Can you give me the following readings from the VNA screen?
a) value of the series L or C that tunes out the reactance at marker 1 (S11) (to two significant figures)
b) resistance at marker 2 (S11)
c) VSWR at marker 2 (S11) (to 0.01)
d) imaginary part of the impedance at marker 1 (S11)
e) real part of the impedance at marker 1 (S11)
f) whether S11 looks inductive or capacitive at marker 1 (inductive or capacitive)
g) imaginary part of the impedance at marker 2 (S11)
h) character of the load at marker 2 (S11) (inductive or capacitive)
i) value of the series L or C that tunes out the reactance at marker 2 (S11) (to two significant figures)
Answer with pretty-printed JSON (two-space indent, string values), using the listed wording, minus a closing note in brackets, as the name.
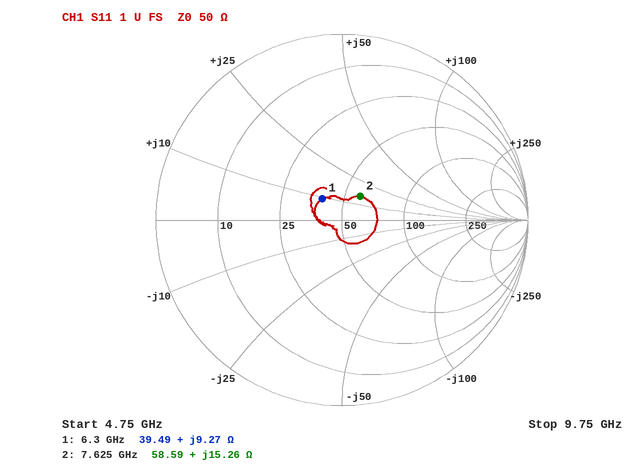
{
  "value of the series L or C that tunes out the reactance at marker 1 (S11)": "2.7 pF",
  "resistance at marker 2": "58.59 Ω",
  "VSWR at marker 2 (S11)": "1.38",
  "imaginary part of the impedance at marker 1": "+9.27 Ω",
  "real part of the impedance at marker 1": "39.49 Ω",
  "whether S11 looks inductive or capacitive at marker 1": "inductive",
  "imaginary part of the impedance at marker 2": "+15.26 Ω",
  "character of the load at marker 2 (S11)": "inductive",
  "value of the series L or C that tunes out the reactance at marker 2 (S11)": "1.4 pF"
}
